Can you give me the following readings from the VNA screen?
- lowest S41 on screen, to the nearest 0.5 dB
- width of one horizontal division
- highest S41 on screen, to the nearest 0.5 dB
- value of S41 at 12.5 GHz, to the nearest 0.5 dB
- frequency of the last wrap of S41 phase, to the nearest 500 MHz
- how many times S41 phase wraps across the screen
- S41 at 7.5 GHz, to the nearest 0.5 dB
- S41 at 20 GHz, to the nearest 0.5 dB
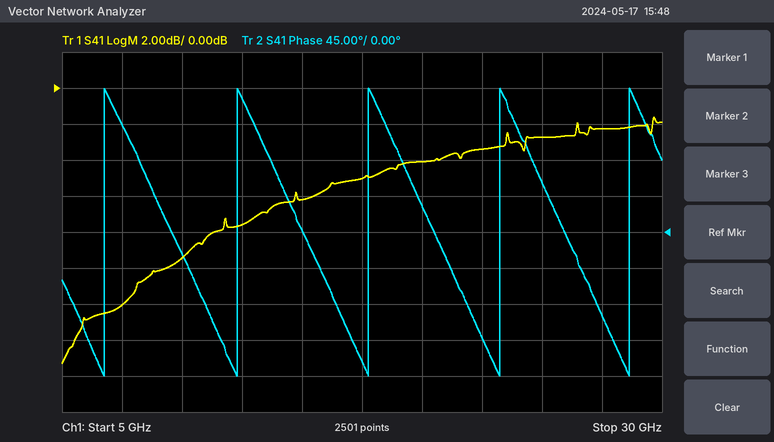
-15.5 dB
2.5 GHz
-1.5 dB
-7.5 dB
28.5 GHz
5
-12.0 dB
-4.0 dB
